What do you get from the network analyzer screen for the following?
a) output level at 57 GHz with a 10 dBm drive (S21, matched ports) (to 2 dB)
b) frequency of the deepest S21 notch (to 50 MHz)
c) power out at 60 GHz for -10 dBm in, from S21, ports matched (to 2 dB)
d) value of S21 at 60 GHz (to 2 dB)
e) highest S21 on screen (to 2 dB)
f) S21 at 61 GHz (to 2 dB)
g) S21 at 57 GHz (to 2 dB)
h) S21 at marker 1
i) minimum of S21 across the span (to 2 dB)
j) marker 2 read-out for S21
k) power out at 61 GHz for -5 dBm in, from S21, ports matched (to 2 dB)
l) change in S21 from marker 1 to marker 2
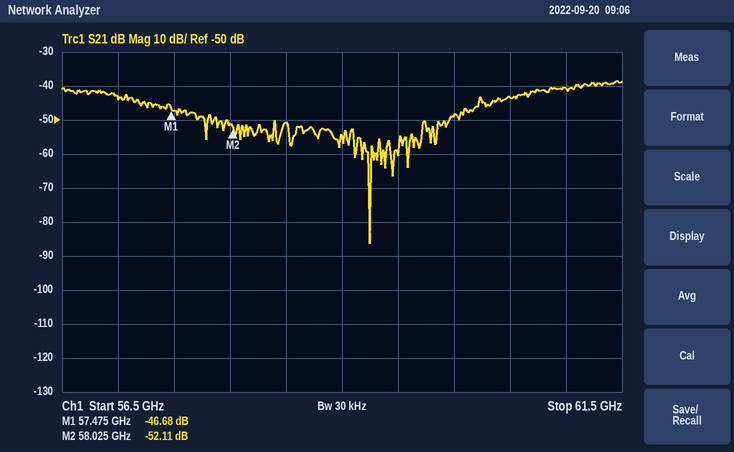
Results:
-34 dBm
59.25 GHz
-58 dBm
-48 dB
-38 dB
-40 dB
-44 dB
-46.68 dB
-86 dB
-52.11 dB
-46 dBm
-5.43 dB
